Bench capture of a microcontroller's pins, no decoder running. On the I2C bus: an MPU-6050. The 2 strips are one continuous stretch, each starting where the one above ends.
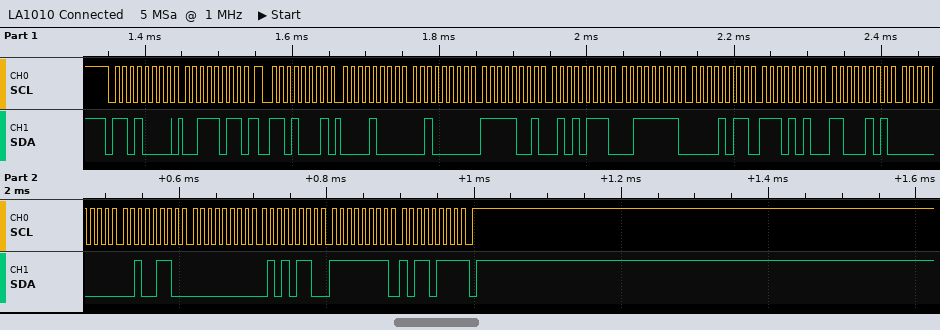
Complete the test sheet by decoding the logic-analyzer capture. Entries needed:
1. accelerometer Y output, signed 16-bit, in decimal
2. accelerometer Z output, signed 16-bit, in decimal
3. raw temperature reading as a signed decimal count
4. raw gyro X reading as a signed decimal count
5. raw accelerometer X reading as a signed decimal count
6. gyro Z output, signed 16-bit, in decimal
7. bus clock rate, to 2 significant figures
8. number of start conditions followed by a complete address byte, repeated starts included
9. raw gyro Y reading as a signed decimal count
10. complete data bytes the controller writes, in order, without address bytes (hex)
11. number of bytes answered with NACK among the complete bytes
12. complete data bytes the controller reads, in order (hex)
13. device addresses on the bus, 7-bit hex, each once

-1705
16139
-5435
38
2080
-73
100 kHz
2
86
3B
1
08 20 F9 57 3F 0B EA C5 00 26 00 56 FF B7
0x68
